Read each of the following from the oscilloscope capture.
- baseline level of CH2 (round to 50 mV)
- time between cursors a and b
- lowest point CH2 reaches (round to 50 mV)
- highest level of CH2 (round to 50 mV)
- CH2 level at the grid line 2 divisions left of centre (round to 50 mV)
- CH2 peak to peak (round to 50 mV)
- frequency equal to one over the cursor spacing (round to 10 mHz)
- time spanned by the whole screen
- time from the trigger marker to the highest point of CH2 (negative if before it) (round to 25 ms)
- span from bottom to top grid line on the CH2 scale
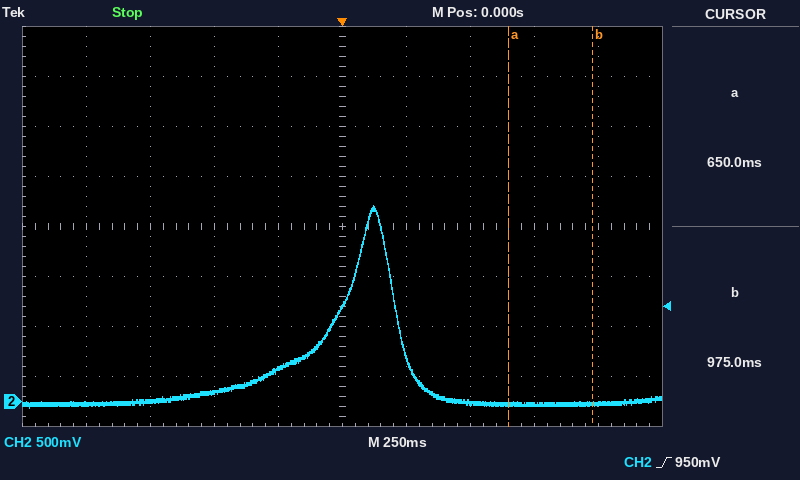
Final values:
0 mV
325 ms
-50 mV
1.95 V
100 mV
2.00 V
3.08 Hz
2.5 s
+125 ms
4 V
